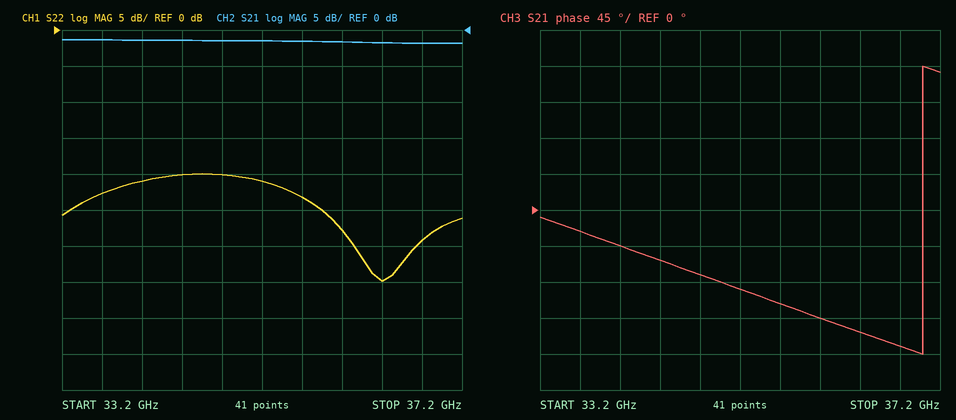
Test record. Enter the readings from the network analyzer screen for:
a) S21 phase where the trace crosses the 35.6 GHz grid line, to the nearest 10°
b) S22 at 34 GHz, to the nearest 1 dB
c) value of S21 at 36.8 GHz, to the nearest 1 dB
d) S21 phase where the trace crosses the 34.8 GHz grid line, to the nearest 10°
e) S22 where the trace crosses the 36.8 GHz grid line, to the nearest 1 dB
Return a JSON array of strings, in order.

["-120°", "-21 dB", "-2 dB", "-80°", "-29 dB"]
